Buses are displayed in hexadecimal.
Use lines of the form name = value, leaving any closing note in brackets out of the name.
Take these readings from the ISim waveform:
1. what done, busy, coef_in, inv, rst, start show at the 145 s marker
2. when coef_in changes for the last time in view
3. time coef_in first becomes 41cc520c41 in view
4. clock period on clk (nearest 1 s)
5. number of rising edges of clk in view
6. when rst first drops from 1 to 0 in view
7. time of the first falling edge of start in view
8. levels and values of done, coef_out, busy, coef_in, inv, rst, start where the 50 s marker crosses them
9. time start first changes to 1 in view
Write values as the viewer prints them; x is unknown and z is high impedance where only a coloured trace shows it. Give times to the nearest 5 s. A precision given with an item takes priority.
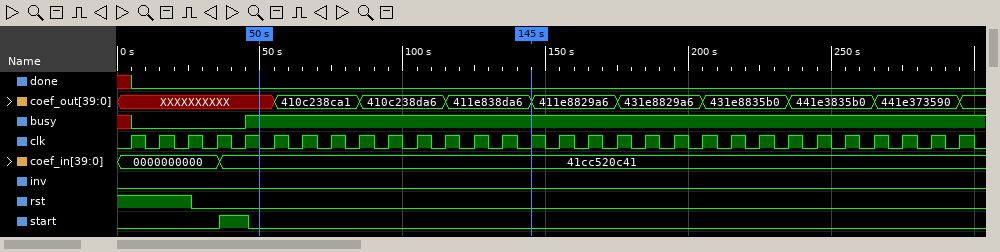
what done, busy, coef_in, inv, rst, start show at the 145 s marker = done=0, busy=1, coef_in=41cc520c41, inv=0, rst=0, start=0
when coef_in changes for the last time in view = 35 s
time coef_in first becomes 41cc520c41 in view = 35 s
clock period on clk = 10 s
number of rising edges of clk in view = 30
when rst first drops from 1 to 0 in view = 25 s
time of the first falling edge of start in view = 45 s
levels and values of done, coef_out, busy, coef_in, inv, rst, start where the 50 s marker crosses them = done=0, coef_out=XXXXXXXXXX, busy=1, coef_in=41cc520c41, inv=0, rst=0, start=0
time start first changes to 1 in view = 35 s
